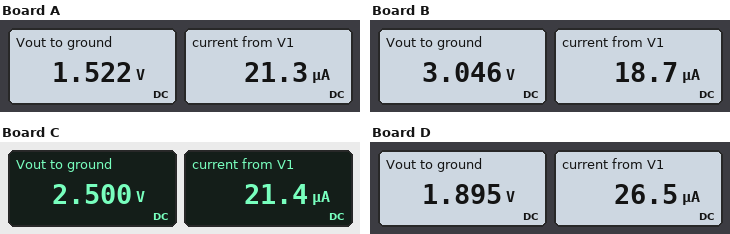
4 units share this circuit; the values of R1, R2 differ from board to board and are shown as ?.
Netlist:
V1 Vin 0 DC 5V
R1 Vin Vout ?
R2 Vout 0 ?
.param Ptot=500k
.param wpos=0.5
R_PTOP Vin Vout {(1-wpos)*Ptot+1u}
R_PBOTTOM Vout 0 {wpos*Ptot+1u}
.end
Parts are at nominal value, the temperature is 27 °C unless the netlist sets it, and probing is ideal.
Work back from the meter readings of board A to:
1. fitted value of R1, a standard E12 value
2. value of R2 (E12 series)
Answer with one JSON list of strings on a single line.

["470 kΩ", "100 kΩ"]
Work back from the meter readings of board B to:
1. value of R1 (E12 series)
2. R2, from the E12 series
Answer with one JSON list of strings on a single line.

["180 kΩ", "470 kΩ"]
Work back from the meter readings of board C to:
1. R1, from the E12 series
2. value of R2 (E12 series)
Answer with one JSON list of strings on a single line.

["220 kΩ", "220 kΩ"]
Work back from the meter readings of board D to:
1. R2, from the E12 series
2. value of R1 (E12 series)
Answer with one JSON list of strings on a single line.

["100 kΩ", "220 kΩ"]
